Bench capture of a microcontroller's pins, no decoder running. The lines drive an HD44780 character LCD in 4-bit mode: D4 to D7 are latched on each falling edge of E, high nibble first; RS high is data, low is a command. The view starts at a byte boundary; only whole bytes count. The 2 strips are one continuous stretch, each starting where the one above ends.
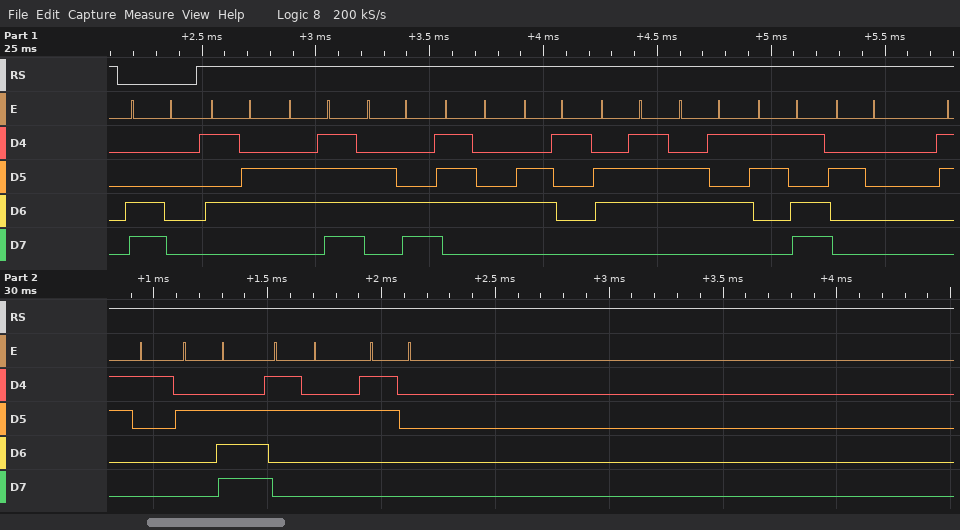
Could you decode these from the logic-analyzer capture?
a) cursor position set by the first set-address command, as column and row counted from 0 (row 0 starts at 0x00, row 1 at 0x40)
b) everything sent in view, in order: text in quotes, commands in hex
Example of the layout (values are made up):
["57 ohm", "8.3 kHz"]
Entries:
["column 0, row 1", "0xC0 \"Voltage= 1.20\""]
